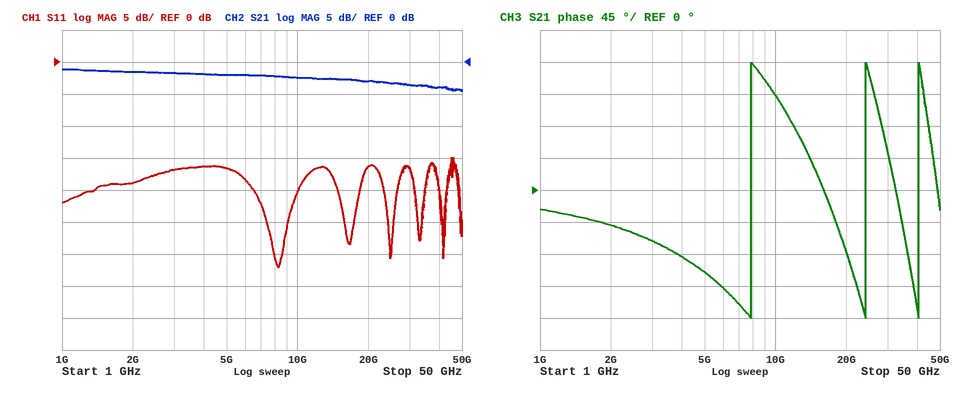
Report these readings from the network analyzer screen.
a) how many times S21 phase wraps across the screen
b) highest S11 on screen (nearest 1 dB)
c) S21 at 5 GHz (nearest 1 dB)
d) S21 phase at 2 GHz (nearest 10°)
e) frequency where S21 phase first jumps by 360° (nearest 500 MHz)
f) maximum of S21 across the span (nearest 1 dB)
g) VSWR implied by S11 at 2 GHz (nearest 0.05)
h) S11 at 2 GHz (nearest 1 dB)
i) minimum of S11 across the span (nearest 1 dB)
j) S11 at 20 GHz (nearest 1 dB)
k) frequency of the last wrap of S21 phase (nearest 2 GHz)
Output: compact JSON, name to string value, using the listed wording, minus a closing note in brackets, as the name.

{"how many times S21 phase wraps across the screen": "3", "highest S11 on screen": "-15 dB", "S21 at 5 GHz": "-2 dB", "S21 phase at 2 GHz": "-50°", "frequency where S21 phase first jumps by 360°": "8.0 GHz", "maximum of S21 across the span": "-1 dB", "VSWR implied by S11 at 2 GHz": "1.25", "S11 at 2 GHz": "-19 dB", "minimum of S11 across the span": "-32 dB", "S11 at 20 GHz": "-16 dB", "frequency of the last wrap of S21 phase": "40 GHz"}
